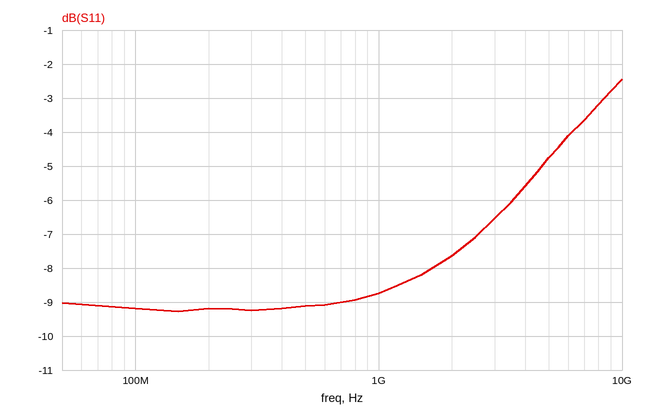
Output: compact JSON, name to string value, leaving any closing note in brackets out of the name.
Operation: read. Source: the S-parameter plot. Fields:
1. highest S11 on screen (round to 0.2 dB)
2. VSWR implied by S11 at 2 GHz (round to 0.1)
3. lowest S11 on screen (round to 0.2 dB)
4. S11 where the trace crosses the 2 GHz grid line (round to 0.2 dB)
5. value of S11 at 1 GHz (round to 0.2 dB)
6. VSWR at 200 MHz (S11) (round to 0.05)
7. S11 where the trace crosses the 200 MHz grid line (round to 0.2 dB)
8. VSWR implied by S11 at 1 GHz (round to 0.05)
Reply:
{"highest S11 on screen": "-2.4 dB", "VSWR implied by S11 at 2 GHz": "2.4", "lowest S11 on screen": "-9.2 dB", "S11 where the trace crosses the 2 GHz grid line": "-7.6 dB", "value of S11 at 1 GHz": "-8.8 dB", "VSWR at 200 MHz (S11)": "2.05", "S11 where the trace crosses the 200 MHz grid line": "-9.2 dB", "VSWR implied by S11 at 1 GHz": "2.15"}
